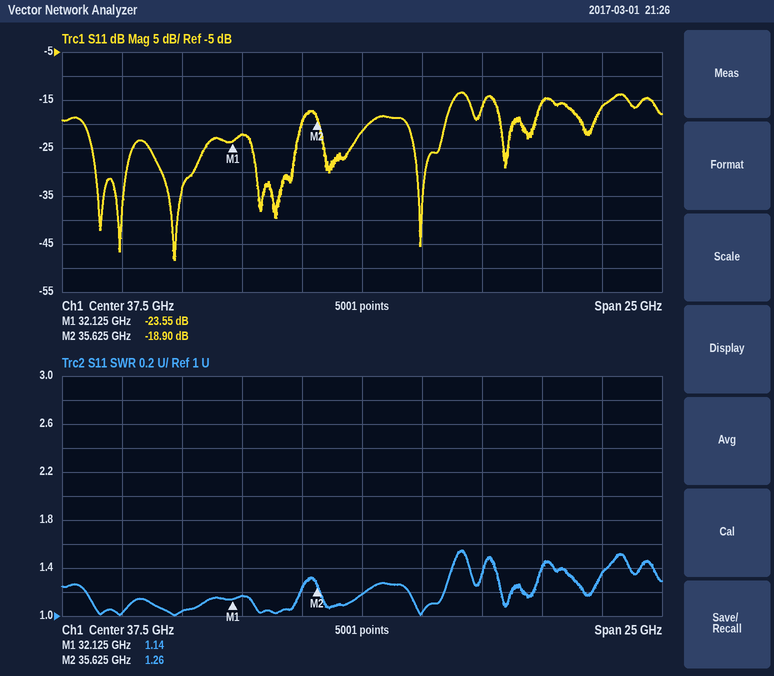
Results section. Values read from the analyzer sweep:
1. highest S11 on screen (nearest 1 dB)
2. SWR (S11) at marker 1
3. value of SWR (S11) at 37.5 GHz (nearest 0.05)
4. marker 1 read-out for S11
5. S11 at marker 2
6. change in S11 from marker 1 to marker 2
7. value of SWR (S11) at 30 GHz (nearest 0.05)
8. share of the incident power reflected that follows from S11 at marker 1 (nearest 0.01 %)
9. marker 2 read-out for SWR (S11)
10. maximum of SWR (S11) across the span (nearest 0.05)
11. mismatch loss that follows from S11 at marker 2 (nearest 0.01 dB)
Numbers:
-13 dB
1.14
1.20
-23.55 dB
-18.90 dB
4.65 dB
1.05
0.44 %
1.26
1.55
0.06 dB
